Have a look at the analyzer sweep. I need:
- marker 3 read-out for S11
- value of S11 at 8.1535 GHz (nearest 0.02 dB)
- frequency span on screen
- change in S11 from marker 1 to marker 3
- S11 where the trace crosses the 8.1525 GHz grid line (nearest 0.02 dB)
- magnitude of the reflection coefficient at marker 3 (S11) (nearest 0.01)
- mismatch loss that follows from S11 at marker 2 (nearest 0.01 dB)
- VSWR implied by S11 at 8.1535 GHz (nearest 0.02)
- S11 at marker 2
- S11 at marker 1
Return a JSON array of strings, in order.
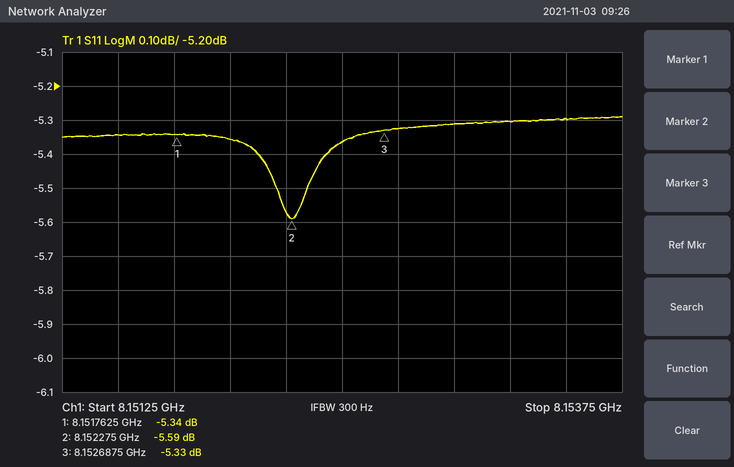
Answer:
["-5.33 dB", "-5.30 dB", "2.5 MHz", "0.01 dB", "-5.36 dB", "0.54", "1.40 dB", "3.38", "-5.59 dB", "-5.34 dB"]
